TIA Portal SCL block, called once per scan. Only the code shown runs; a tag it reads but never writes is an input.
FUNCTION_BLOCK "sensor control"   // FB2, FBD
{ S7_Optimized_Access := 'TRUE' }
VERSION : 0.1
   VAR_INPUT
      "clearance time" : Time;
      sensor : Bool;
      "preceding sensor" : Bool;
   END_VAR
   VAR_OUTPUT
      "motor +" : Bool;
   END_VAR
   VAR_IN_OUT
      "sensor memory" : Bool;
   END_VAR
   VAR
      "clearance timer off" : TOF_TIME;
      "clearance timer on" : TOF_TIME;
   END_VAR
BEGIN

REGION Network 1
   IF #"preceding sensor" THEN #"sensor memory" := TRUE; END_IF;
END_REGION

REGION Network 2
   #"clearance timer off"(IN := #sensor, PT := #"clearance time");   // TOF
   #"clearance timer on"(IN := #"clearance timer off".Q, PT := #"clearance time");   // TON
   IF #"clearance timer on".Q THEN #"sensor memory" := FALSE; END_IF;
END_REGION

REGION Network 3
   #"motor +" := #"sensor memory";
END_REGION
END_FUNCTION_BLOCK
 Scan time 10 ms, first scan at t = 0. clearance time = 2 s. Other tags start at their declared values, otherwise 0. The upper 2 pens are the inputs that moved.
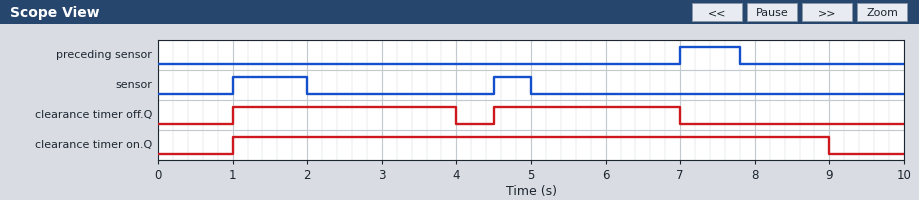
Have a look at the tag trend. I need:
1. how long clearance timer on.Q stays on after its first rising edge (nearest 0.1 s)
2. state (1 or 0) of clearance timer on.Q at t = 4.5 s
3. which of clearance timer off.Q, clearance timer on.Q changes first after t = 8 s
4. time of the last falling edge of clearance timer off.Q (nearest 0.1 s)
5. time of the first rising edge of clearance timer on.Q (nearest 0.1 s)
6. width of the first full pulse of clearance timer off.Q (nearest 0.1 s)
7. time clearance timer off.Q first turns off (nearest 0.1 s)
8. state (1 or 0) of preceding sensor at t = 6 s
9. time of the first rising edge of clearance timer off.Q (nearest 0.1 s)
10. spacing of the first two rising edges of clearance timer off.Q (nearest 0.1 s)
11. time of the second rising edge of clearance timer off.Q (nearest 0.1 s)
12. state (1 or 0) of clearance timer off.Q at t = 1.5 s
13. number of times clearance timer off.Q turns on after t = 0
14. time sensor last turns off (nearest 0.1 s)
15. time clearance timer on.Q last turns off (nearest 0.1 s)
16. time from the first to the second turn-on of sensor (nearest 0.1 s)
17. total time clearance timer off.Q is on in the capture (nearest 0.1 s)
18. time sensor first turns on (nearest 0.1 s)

8.0 s
1
clearance timer on.Q
7.0 s
1.0 s
3.0 s
4.0 s
0
1.0 s
3.5 s
4.5 s
1
2
5.0 s
9.0 s
3.5 s
5.5 s
1.0 s
